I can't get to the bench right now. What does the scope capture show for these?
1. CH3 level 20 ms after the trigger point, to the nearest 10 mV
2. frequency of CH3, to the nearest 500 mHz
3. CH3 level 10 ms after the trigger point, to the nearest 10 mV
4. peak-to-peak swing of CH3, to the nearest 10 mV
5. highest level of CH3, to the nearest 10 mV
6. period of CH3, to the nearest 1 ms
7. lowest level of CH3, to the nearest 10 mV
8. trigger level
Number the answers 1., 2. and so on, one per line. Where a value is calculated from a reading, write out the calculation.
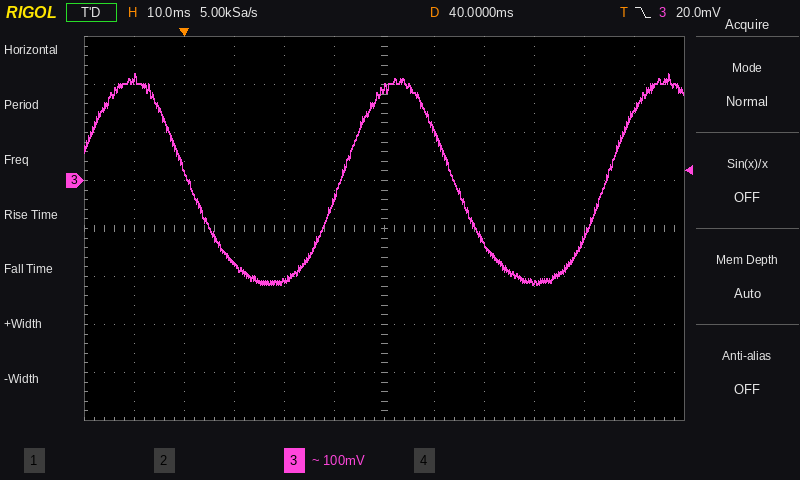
1. -210 mV
2. 1 / 53 ms ≈ 18.9 Hz, so 19.0 Hz to the nearest 500 mHz
3. -170 mV
4. 220 mV − (-220 mV) = 440 mV
5. 220 mV
6. 53 ms
7. -220 mV
8. 20.0 mV
